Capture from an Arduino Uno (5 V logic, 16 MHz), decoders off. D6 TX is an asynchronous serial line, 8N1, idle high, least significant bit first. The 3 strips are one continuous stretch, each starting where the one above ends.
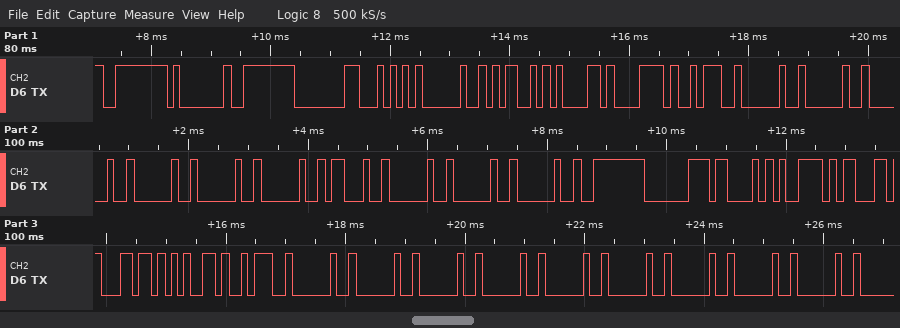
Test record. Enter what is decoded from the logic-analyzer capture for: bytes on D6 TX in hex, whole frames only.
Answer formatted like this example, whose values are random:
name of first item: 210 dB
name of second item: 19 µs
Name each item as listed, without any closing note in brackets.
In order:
bytes on D6 TX in hex, whole frames only: FE 01 FE 80 54 20 4D 61 78 3A 20 20 20 20 20 20 23 20 20 20 FE C0 43 79 63 6C 65 3A 20 20 20 20 20 20 20 20 20
